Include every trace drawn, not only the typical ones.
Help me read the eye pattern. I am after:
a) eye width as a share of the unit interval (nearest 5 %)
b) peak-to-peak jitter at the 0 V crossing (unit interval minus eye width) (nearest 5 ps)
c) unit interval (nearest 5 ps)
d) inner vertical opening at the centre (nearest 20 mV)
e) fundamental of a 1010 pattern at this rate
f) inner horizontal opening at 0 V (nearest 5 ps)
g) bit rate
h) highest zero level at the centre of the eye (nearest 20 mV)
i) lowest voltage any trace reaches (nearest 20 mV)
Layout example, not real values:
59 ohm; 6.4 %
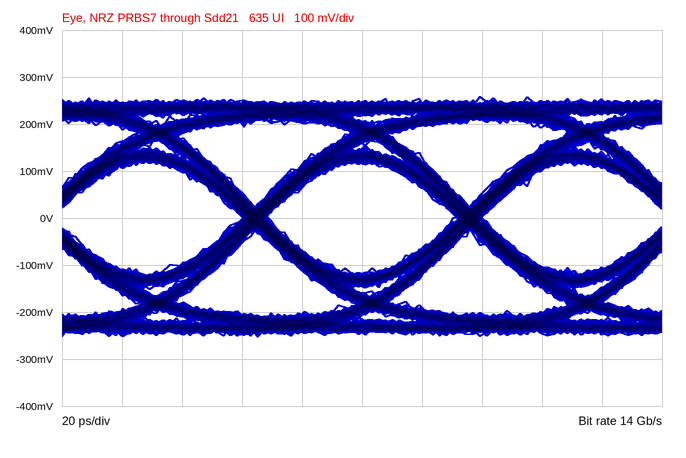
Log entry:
85 %; 10 ps; 70 ps; 240 mV; 7 GHz; 60 ps; 14 Gb/s; -120 mV; -260 mV
